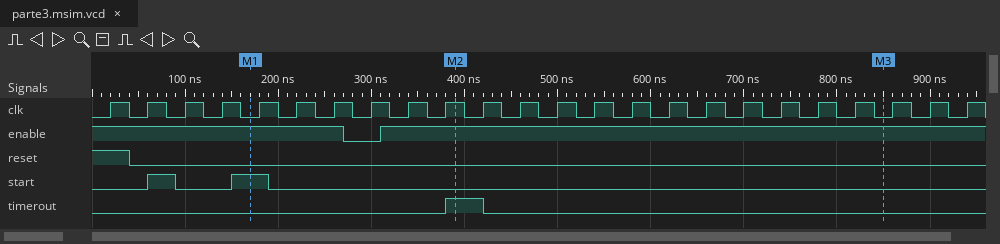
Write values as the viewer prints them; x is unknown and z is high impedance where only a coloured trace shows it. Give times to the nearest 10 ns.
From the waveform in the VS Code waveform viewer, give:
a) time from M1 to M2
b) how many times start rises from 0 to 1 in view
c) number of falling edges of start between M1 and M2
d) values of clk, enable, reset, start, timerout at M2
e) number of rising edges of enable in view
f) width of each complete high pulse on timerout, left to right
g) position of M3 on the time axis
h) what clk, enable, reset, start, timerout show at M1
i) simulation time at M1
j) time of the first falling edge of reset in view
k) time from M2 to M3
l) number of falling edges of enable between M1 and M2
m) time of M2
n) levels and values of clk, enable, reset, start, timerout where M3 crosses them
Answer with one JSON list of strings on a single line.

["220 ns", "2", "1", "clk=1, enable=1, reset=0, start=0, timerout=1", "1", "40 ns", "850 ns", "clk=0, enable=1, reset=0, start=1, timerout=0", "170 ns", "40 ns", "460 ns", "1", "390 ns", "clk=0, enable=1, reset=0, start=0, timerout=0"]
